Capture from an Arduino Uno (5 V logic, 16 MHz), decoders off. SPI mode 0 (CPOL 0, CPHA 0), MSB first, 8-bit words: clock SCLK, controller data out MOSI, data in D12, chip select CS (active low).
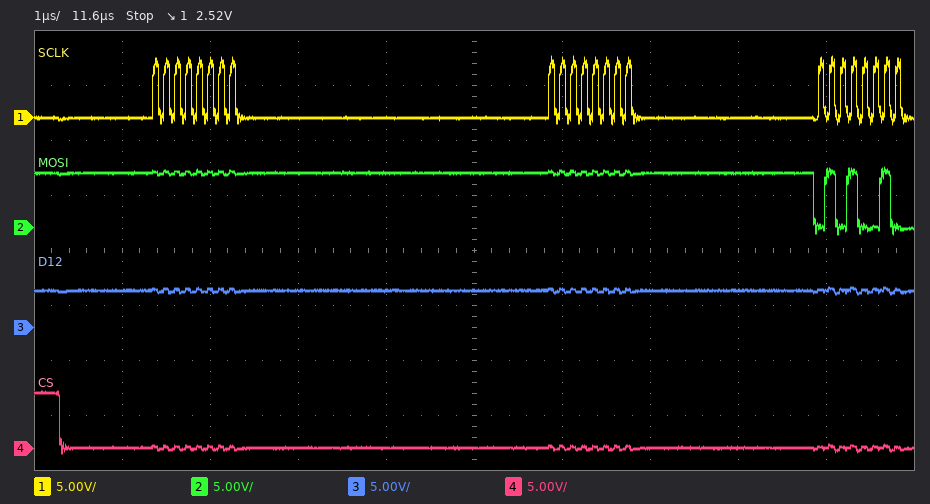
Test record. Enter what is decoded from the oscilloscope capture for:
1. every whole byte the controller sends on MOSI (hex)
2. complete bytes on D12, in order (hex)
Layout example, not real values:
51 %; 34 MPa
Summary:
FF FF 52; FF FF FF
